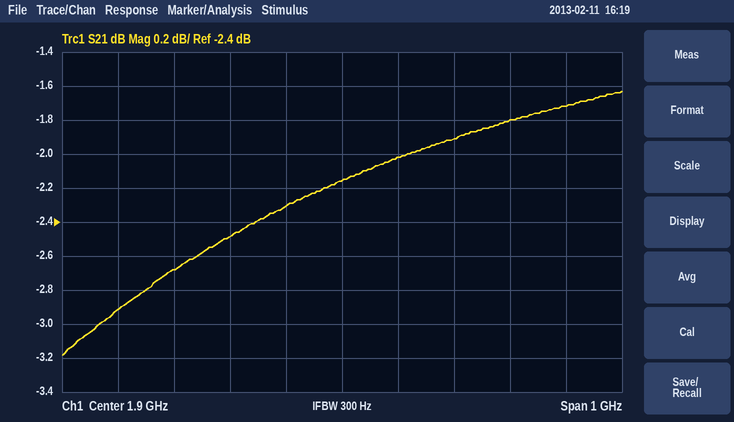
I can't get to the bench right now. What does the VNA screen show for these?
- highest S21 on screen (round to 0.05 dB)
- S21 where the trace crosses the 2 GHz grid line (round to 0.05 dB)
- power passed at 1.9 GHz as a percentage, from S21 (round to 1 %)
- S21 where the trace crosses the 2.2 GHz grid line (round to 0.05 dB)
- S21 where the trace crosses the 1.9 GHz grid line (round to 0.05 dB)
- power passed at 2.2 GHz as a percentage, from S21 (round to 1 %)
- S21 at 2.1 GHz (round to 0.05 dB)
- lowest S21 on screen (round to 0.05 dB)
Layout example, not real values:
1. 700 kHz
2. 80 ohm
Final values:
1. -1.65 dB
2. -2.00 dB
3. 61 %
4. -1.80 dB
5. -2.15 dB
6. 66 %
7. -1.90 dB
8. -3.20 dB
